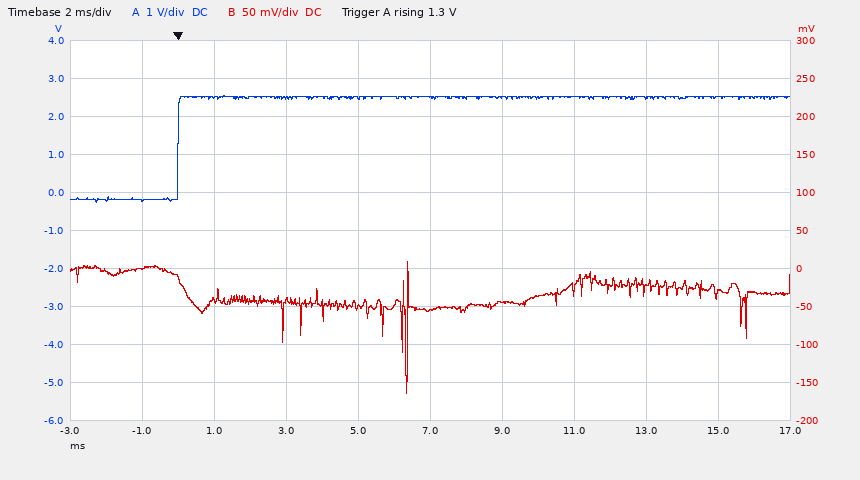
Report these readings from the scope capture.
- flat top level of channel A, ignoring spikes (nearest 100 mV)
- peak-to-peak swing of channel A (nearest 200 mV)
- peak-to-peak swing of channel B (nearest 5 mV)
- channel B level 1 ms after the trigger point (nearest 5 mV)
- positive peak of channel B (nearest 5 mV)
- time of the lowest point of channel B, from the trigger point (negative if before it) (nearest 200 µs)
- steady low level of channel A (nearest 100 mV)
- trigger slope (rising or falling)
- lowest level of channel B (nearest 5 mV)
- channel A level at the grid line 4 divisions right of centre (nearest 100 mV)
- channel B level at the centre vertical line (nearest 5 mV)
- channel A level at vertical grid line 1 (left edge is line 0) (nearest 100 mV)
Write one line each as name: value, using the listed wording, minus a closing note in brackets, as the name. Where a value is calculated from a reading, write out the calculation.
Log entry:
flat top level of channel A, ignoring spikes: 2.5 V
peak-to-peak swing of channel A: 2.8 V
peak-to-peak swing of channel B: 10 mV − (-165 mV) = 175 mV
channel B level 1 ms after the trigger point: -40 mV
positive peak of channel B: 10 mV
time of the lowest point of channel B, from the trigger point (negative if before it): +6.4 ms
steady low level of channel A: -200 mV
trigger slope: rising
lowest level of channel B: -165 mV
channel A level at the grid line 4 divisions right of centre: 2.5 V
channel B level at the centre vertical line: -55 mV
channel A level at vertical grid line 1 (left edge is line 0): -200 mV
